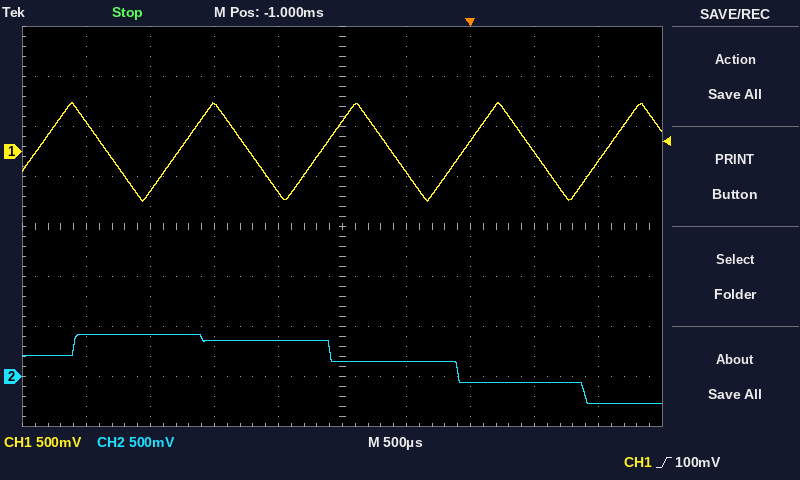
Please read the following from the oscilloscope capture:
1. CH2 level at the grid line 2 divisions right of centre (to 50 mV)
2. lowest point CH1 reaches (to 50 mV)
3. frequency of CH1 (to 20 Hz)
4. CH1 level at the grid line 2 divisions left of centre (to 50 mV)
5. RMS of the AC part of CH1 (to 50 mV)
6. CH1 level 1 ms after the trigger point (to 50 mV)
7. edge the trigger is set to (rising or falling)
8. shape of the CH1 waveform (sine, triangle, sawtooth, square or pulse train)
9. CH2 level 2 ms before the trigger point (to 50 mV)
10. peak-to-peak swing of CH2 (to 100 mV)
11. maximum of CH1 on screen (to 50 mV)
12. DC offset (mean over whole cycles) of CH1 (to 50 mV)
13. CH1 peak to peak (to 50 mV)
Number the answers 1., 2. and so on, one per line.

1. -50 mV
2. -500 mV
3. 900 Hz
4. 450 mV
5. 300 mV
6. -100 mV
7. rising
8. triangle
9. 350 mV
10. 700 mV
11. 500 mV
12. 0 mV
13. 1.00 V
